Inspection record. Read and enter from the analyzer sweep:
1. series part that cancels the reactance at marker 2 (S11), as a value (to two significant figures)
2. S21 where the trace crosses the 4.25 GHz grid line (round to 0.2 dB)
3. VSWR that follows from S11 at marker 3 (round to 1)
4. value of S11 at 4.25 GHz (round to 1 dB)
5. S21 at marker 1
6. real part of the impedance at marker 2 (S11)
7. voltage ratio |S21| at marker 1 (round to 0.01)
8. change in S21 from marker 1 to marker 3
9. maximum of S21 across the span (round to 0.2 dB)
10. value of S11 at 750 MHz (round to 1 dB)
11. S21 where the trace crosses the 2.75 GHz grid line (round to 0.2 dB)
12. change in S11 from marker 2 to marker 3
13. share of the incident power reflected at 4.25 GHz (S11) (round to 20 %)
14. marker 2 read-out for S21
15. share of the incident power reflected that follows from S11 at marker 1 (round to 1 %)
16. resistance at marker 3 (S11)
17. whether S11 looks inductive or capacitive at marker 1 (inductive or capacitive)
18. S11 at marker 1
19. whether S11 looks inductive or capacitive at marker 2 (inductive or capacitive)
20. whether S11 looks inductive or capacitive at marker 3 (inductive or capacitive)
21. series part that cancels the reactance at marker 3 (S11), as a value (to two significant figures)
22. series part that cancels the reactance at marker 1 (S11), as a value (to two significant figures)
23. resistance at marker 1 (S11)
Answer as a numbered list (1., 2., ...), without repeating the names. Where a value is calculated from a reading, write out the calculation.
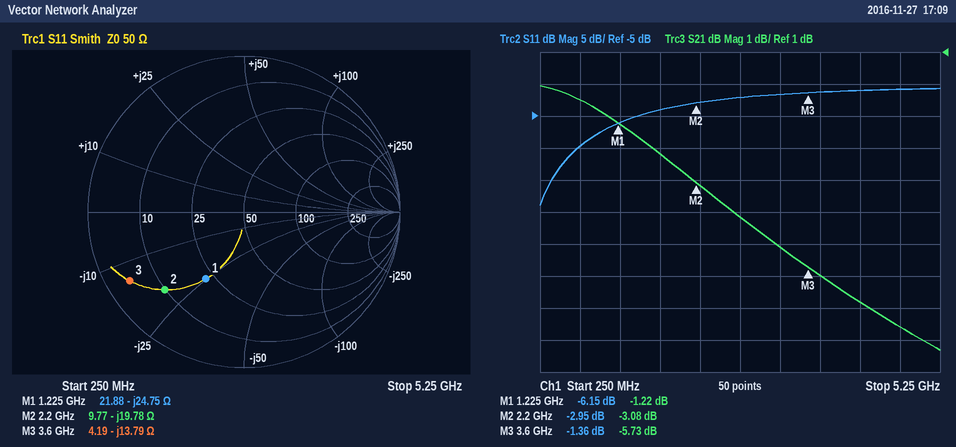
1. L = 19.78 Ω/(2π × 2.2 GHz) ≈ 1.4 nH
2. -6.8 dB
3. (1 + 0.8551)/(1 − 0.8551) ≈ 13
4. -1 dB
5. -1.22 dB
6. 9.77 Ω
7. 10^(-1.22/20) ≈ 0.87
8. -5.73 − (-1.22) = -4.51 dB
9. 0.0 dB
10. -10 dB
11. -4.2 dB
12. -1.36 − (-2.95) = 1.59 dB
13. 10^(-1/10) ≈ 79.4 %, so 80 % to the nearest 20 %
14. -3.08 dB
15. 10^(-6.15/10) ≈ 24 %
16. 4.19 Ω
17. capacitive
18. -6.15 dB
19. capacitive
20. capacitive
21. L = 13.79 Ω/(2π × 3.6 GHz) ≈ 610 pH
22. L = 24.75 Ω/(2π × 1.225 GHz) ≈ 3.2 nH
23. 21.88 Ω
